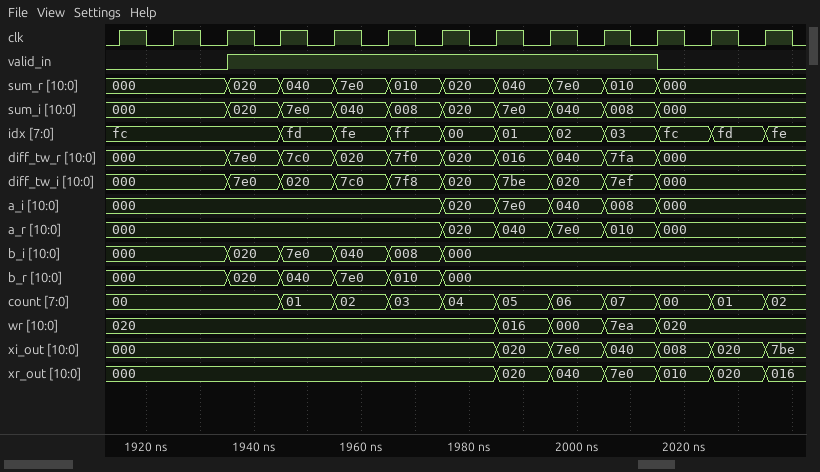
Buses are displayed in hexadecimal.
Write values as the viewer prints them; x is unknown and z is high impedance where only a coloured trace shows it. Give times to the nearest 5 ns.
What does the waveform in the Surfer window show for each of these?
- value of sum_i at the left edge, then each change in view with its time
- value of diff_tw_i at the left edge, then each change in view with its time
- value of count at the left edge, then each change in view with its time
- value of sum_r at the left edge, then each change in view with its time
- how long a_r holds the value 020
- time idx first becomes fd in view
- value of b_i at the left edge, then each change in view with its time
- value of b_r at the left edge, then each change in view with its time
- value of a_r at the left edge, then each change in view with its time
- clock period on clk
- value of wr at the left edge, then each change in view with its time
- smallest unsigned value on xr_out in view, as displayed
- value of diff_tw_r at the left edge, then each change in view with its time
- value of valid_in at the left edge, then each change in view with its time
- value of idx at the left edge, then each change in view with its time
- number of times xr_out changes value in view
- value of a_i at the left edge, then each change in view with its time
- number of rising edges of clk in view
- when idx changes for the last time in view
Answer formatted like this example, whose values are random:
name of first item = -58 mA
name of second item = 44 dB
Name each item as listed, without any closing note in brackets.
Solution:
value of sum_i at the left edge, then each change in view with its time = 000, 020 at 1935 ns, 7e0 at 1945 ns, 040 at 1955 ns, 008 at 1965 ns, 020 at 1975 ns, 7e0 at 1985 ns, 040 at 1995 ns, 008 at 2005 ns, 000 at 2015 ns
value of diff_tw_i at the left edge, then each change in view with its time = 000, 7e0 at 1935 ns, 020 at 1945 ns, 7c0 at 1955 ns, 7f8 at 1965 ns, 020 at 1975 ns, 7be at 1985 ns, 020 at 1995 ns, 7ef at 2005 ns, 000 at 2015 ns
value of count at the left edge, then each change in view with its time = 00, 01 at 1945 ns, 02 at 1955 ns, 03 at 1965 ns, 04 at 1975 ns, 05 at 1985 ns, 06 at 1995 ns, 07 at 2005 ns, 00 at 2015 ns, 01 at 2025 ns, 02 at 2035 ns
value of sum_r at the left edge, then each change in view with its time = 000, 020 at 1935 ns, 040 at 1945 ns, 7e0 at 1955 ns, 010 at 1965 ns, 020 at 1975 ns, 040 at 1985 ns, 7e0 at 1995 ns, 010 at 2005 ns, 000 at 2015 ns
how long a_r holds the value 020 = 10 ns
time idx first becomes fd in view = 1945 ns
value of b_i at the left edge, then each change in view with its time = 000, 020 at 1935 ns, 7e0 at 1945 ns, 040 at 1955 ns, 008 at 1965 ns, 000 at 1975 ns
value of b_r at the left edge, then each change in view with its time = 000, 020 at 1935 ns, 040 at 1945 ns, 7e0 at 1955 ns, 010 at 1965 ns, 000 at 1975 ns
value of a_r at the left edge, then each change in view with its time = 000, 020 at 1975 ns, 040 at 1985 ns, 7e0 at 1995 ns, 010 at 2005 ns, 000 at 2015 ns
clock period on clk = 10 ns
value of wr at the left edge, then each change in view with its time = 020, 016 at 1985 ns, 000 at 1995 ns, 7ea at 2005 ns, 020 at 2015 ns
smallest unsigned value on xr_out in view, as displayed = 000
value of diff_tw_r at the left edge, then each change in view with its time = 000, 7e0 at 1935 ns, 7c0 at 1945 ns, 020 at 1955 ns, 7f0 at 1965 ns, 020 at 1975 ns, 016 at 1985 ns, 040 at 1995 ns, 7fa at 2005 ns, 000 at 2015 ns
value of valid_in at the left edge, then each change in view with its time = 0, 1 at 1935 ns, 0 at 2015 ns
value of idx at the left edge, then each change in view with its time = fc, fd at 1945 ns, fe at 1955 ns, ff at 1965 ns, 00 at 1975 ns, 01 at 1985 ns, 02 at 1995 ns, 03 at 2005 ns, fc at 2015 ns, fd at 2025 ns, fe at 2035 ns
number of times xr_out changes value in view = 6
value of a_i at the left edge, then each change in view with its time = 000, 020 at 1975 ns, 7e0 at 1985 ns, 040 at 1995 ns, 008 at 2005 ns, 000 at 2015 ns
number of rising edges of clk in view = 13
when idx changes for the last time in view = 2035 ns
